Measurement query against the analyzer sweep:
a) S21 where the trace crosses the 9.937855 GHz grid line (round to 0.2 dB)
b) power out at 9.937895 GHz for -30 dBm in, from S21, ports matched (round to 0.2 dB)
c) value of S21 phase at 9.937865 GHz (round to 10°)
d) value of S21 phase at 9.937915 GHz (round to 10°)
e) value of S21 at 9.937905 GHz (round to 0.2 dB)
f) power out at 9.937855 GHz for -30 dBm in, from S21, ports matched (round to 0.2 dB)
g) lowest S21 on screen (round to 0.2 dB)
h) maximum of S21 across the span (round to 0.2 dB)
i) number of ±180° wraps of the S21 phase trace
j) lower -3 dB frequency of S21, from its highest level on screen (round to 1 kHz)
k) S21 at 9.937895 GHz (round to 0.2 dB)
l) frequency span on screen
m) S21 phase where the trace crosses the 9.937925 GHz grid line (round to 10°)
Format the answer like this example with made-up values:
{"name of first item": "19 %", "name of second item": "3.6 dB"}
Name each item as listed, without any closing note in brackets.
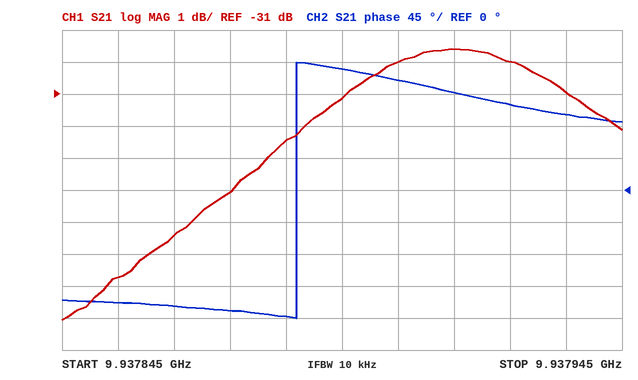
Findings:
{"S21 where the trace crosses the 9.937855 GHz grid line": "-36.8 dB", "power out at 9.937895 GHz for -30 dBm in, from S21, ports matched": "-61.2 dBm", "value of S21 phase at 9.937865 GHz": "-160°", "value of S21 phase at 9.937915 GHz": "140°", "value of S21 at 9.937905 GHz": "-30.0 dB", "power out at 9.937855 GHz for -30 dBm in, from S21, ports matched": "-66.8 dBm", "lowest S21 on screen": "-38.0 dB", "maximum of S21 across the span": "-29.6 dB", "number of ±180° wraps of the S21 phase trace": "1", "lower -3 dB frequency of S21, from its highest level on screen": "9.937884 GHz", "S21 at 9.937895 GHz": "-31.2 dB", "frequency span on screen": "100 kHz", "S21 phase where the trace crosses the 9.937925 GHz grid line": "120°"}
